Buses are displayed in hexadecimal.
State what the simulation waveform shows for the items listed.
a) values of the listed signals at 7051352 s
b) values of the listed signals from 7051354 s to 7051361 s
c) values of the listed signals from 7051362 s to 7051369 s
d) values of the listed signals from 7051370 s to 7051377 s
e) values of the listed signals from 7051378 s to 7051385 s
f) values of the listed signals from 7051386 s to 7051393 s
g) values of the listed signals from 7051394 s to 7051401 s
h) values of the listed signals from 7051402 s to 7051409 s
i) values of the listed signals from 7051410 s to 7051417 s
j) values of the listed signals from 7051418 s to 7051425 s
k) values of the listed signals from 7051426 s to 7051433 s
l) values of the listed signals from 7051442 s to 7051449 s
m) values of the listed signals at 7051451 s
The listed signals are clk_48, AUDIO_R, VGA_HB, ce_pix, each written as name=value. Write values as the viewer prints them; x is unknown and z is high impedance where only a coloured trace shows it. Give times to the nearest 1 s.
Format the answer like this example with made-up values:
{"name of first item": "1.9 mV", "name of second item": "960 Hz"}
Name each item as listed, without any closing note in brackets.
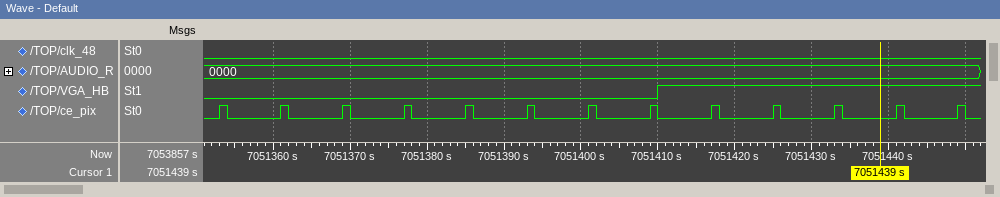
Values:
{"values of the listed signals at 7051352 s": "clk_48=0, AUDIO_R=0000, VGA_HB=0, ce_pix=0", "values of the listed signals from 7051354 s to 7051361 s": "clk_48=0, AUDIO_R=0000, VGA_HB=0, ce_pix=0", "values of the listed signals from 7051362 s to 7051369 s": "clk_48=0, AUDIO_R=0000, VGA_HB=0, ce_pix=0", "values of the listed signals from 7051370 s to 7051377 s": "clk_48=0, AUDIO_R=0000, VGA_HB=0, ce_pix=0", "values of the listed signals from 7051378 s to 7051385 s": "clk_48=0, AUDIO_R=0000, VGA_HB=0, ce_pix=0", "values of the listed signals from 7051386 s to 7051393 s": "clk_48=0, AUDIO_R=0000, VGA_HB=0, ce_pix=0", "values of the listed signals from 7051394 s to 7051401 s": "clk_48=0, AUDIO_R=0000, VGA_HB=0, ce_pix=0", "values of the listed signals from 7051402 s to 7051409 s": "clk_48=0, AUDIO_R=0000, VGA_HB=0, ce_pix=0", "values of the listed signals from 7051410 s to 7051417 s": "clk_48=0, AUDIO_R=0000, VGA_HB=1, ce_pix=0", "values of the listed signals from 7051418 s to 7051425 s": "clk_48=0, AUDIO_R=0000, VGA_HB=1, ce_pix=0", "values of the listed signals from 7051426 s to 7051433 s": "clk_48=0, AUDIO_R=0000, VGA_HB=1, ce_pix=0", "values of the listed signals from 7051442 s to 7051449 s": "clk_48=0, AUDIO_R=0000, VGA_HB=1, ce_pix=0", "values of the listed signals at 7051451 s": "clk_48=0, AUDIO_R=0000, VGA_HB=1, ce_pix=0"}
